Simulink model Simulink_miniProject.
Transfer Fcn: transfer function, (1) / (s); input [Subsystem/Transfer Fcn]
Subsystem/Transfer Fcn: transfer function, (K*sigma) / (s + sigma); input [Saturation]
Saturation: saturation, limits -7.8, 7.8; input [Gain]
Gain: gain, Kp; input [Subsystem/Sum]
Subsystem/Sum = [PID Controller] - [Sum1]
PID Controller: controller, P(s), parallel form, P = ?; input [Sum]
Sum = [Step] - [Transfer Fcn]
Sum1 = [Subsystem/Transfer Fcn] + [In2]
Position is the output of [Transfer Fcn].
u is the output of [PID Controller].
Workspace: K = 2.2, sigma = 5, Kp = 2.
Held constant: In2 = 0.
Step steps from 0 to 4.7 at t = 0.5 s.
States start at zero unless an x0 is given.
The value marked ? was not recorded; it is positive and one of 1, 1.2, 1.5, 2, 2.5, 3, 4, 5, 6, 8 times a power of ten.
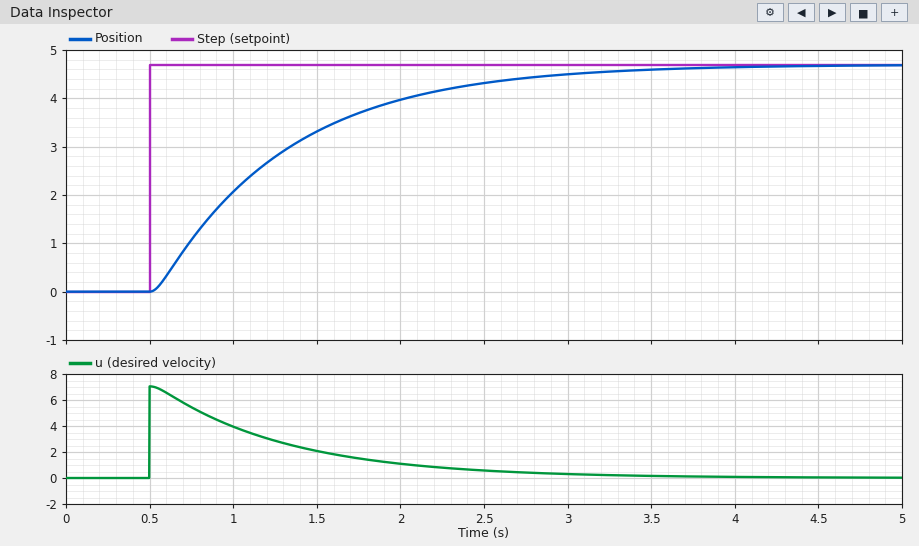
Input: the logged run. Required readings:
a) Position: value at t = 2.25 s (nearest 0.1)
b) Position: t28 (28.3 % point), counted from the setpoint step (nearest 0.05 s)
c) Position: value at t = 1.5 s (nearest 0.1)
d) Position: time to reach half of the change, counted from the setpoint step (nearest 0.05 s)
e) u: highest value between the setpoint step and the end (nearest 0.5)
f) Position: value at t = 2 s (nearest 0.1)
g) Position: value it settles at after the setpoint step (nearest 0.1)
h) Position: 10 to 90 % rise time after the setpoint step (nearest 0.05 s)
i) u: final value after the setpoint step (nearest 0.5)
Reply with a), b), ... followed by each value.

a) 4.2
b) 0.30 s
c) 3.3
d) 0.60 s
e) 7.0
f) 4.0
g) 4.7
h) 1.70 s
i) 0.0
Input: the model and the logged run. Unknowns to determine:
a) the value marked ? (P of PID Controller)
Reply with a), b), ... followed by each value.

a) 1.5
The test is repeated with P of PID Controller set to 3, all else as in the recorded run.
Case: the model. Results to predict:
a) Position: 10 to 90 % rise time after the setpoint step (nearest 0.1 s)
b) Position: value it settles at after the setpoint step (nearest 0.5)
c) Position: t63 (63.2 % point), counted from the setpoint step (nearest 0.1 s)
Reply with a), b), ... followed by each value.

a) 0.8 s
b) 4.5
c) 0.5 s
